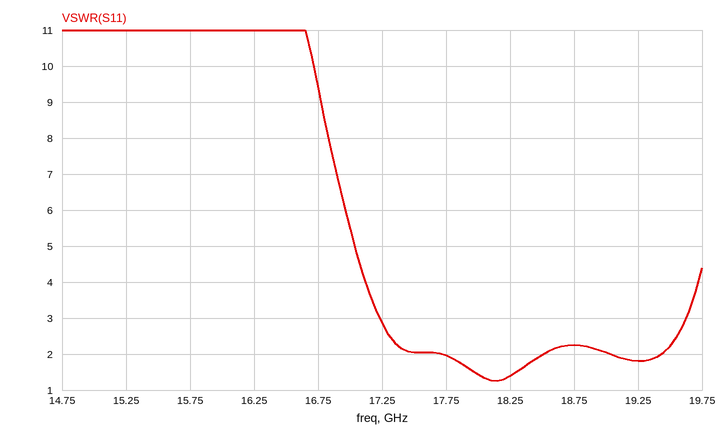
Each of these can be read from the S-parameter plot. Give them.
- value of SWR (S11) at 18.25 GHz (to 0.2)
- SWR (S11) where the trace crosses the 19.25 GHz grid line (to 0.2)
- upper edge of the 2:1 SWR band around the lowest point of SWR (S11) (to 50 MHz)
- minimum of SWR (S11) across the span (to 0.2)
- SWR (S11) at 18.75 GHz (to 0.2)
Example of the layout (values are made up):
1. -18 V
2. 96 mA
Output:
1. 1.4
2. 1.8
3. 18.50 GHz
4. 1.2
5. 2.2
